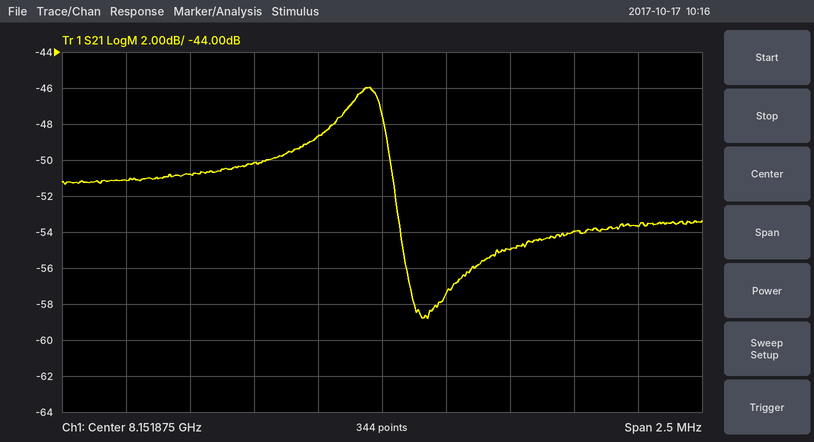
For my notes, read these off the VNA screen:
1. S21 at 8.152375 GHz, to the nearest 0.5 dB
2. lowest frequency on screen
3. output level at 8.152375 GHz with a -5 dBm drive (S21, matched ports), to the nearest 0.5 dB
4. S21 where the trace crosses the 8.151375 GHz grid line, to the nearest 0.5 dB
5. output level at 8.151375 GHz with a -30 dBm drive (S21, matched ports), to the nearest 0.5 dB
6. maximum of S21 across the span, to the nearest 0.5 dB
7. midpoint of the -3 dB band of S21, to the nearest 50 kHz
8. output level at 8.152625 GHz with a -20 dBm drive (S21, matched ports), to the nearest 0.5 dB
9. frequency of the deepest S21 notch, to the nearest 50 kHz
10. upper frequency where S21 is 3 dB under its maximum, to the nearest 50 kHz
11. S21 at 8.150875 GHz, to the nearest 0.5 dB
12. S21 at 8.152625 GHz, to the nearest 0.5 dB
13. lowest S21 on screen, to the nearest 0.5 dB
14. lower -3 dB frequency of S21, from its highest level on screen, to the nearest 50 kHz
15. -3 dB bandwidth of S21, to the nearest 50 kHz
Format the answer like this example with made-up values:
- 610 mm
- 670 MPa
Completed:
- -55.0 dB
- 8.150625 GHz
- -60.0 dBm
- -50.0 dB
- -80.0 dBm
- -46.0 dB
- 8.15175 GHz
- -74.0 dBm
- 8.15205 GHz
- 8.15190 GHz
- -51.0 dB
- -54.0 dB
- -59.0 dB
- 8.15160 GHz
- 300 kHz
